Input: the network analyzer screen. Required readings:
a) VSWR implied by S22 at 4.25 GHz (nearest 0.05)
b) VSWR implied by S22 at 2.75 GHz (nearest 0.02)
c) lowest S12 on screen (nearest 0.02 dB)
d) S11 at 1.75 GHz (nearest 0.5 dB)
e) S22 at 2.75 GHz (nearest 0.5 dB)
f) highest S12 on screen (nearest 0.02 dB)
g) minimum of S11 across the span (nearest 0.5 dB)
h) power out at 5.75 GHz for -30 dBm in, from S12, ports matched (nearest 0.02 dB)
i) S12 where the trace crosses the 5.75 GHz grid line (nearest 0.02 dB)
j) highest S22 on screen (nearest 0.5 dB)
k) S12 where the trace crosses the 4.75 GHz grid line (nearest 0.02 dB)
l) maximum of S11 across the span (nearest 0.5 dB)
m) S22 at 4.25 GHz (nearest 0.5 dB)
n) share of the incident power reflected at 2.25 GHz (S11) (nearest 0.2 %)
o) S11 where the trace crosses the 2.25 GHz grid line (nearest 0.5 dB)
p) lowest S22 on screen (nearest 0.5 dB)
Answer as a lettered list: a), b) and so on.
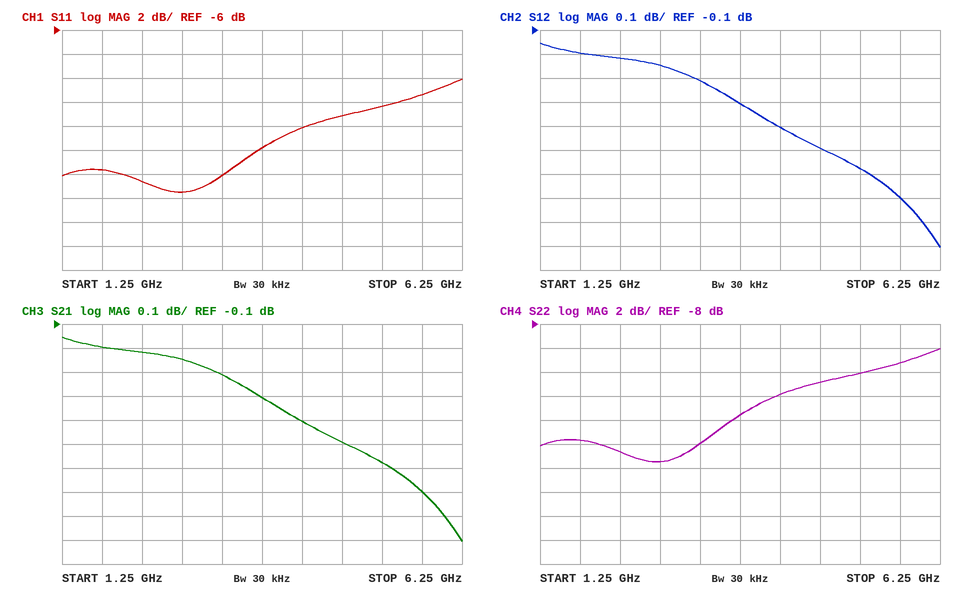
a) 1.50
b) 1.24
c) -1.00 dB
d) -17.5 dB
e) -19.5 dB
f) -0.16 dB
g) -19.5 dB
h) -30.80 dBm
i) -0.80 dB
j) -10.0 dB
k) -0.60 dB
l) -10.0 dB
m) -14.0 dB
n) 1.4 %
o) -18.5 dB
p) -19.5 dB
